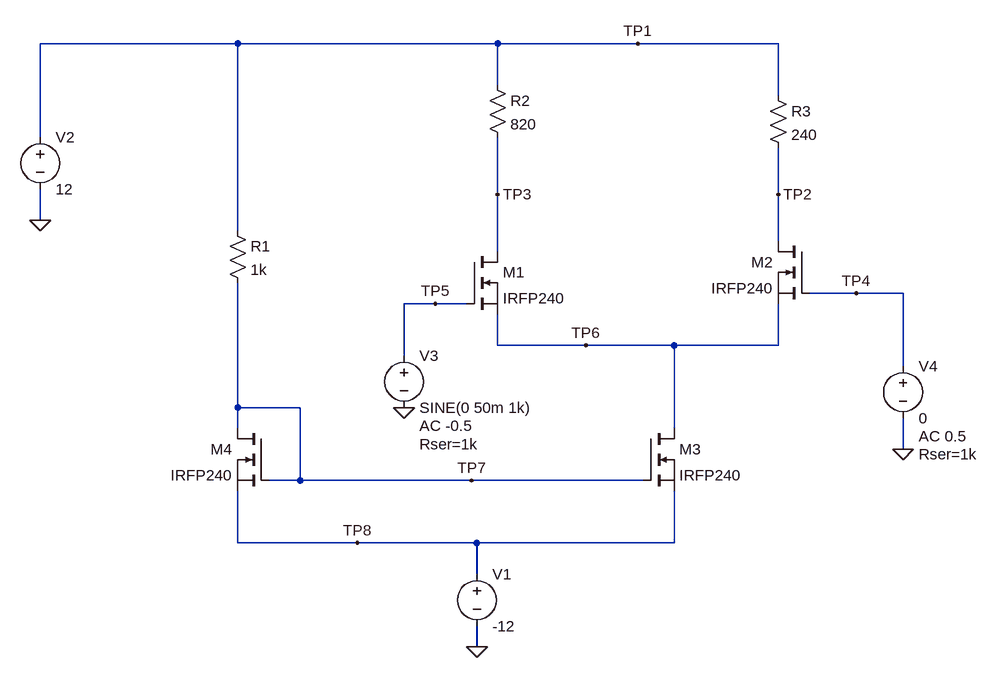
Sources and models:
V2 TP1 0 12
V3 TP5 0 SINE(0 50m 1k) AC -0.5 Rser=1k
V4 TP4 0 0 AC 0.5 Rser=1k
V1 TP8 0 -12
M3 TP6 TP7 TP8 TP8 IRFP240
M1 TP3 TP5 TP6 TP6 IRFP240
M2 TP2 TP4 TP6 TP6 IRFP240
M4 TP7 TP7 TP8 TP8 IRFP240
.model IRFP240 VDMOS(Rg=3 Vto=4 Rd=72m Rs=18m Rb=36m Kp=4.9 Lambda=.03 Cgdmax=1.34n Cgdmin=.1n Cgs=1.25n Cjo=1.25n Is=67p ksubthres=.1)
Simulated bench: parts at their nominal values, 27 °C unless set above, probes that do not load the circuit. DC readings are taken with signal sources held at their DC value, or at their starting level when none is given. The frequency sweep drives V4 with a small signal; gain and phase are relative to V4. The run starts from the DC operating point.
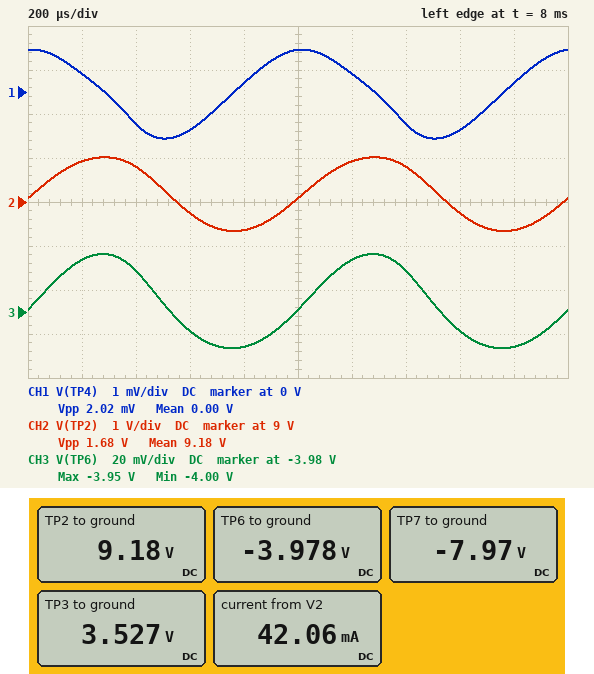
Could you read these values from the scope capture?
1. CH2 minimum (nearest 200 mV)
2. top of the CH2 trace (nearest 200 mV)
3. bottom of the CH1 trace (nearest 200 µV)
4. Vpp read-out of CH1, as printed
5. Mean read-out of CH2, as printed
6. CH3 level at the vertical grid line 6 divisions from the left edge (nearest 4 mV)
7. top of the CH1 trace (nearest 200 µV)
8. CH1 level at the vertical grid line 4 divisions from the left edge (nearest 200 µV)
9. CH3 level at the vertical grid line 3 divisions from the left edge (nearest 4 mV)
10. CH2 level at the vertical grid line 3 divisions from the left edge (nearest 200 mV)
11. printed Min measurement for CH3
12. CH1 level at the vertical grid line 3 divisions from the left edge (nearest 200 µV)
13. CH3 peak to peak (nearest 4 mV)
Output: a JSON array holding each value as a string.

["8.4 V", "10.0 V", "-1.0 mV", "2.02 mV", "9.18 V", "-3.956 V", "1.0 mV", "200 µV", "-3.988 V", "8.8 V", "-4.00 V", "-800 µV", "44 mV"]
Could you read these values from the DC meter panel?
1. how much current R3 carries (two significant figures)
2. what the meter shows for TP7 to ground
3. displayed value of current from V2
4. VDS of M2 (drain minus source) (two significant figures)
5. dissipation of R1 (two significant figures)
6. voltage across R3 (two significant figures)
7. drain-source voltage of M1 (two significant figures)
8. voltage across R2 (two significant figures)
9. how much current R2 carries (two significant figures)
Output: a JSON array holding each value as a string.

["12 mA", "-7.97 V", "42.06 mA", "13 V", "400 mW", "2.8 V", "7.5 V", "8.5 V", "10 mA"]
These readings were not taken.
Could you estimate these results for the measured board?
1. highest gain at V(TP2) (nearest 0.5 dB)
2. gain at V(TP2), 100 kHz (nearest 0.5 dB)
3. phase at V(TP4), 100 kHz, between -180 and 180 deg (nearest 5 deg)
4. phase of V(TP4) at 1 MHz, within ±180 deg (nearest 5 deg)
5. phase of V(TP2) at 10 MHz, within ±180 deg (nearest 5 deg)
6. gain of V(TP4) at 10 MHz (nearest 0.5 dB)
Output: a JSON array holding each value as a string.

["28.5 dB", "7.0 dB", "-10 deg", "-100 deg", "35 deg", "-36.0 dB"]
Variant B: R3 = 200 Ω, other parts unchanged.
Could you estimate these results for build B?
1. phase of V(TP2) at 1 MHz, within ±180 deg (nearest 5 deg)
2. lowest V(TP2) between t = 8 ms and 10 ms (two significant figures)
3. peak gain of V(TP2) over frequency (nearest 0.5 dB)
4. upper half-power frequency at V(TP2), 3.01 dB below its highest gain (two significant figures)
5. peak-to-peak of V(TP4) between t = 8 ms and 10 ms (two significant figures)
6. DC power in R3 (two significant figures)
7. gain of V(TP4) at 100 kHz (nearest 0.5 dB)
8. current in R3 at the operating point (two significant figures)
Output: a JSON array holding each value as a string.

["125 deg", "8.9 V", "27.0 dB", "8.9 kHz", "1.7 mV", "28 mW", "-2.0 dB", "12 mA"]
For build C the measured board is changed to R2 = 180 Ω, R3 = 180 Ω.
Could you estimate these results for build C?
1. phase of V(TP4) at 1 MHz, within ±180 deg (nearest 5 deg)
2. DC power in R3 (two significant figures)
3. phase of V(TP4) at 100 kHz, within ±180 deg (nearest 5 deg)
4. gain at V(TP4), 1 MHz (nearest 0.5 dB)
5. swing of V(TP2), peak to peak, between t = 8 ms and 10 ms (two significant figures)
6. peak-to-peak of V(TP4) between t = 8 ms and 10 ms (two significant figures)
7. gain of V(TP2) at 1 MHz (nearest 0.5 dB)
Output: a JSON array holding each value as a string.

["-70 deg", "22 mW", "-35 deg", "-12.5 dB", "1.4 V", "1.7 mV", "-4.5 dB"]
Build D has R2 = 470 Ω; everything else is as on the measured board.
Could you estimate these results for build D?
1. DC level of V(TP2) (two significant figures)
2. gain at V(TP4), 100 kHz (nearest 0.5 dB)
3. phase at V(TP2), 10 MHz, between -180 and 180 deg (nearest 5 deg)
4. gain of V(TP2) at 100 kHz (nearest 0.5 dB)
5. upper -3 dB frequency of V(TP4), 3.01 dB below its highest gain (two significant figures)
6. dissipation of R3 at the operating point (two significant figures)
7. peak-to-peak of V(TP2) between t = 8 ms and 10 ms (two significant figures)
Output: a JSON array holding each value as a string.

["9.3 V", "-5.5 dB", "30 deg", "12.5 dB", "22 kHz", "31 mW", "1.8 V"]
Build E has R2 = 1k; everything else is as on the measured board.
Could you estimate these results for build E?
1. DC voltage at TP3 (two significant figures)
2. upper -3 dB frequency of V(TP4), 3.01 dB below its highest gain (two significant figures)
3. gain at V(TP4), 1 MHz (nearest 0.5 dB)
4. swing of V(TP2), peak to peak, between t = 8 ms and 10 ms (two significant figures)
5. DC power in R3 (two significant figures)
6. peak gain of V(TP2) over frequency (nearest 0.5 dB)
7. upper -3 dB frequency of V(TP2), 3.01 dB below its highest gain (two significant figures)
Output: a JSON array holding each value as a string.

["1.9 V", "690 kHz", "-7.0 dB", "1.6 V", "34 mW", "28.0 dB", "5.6 kHz"]
